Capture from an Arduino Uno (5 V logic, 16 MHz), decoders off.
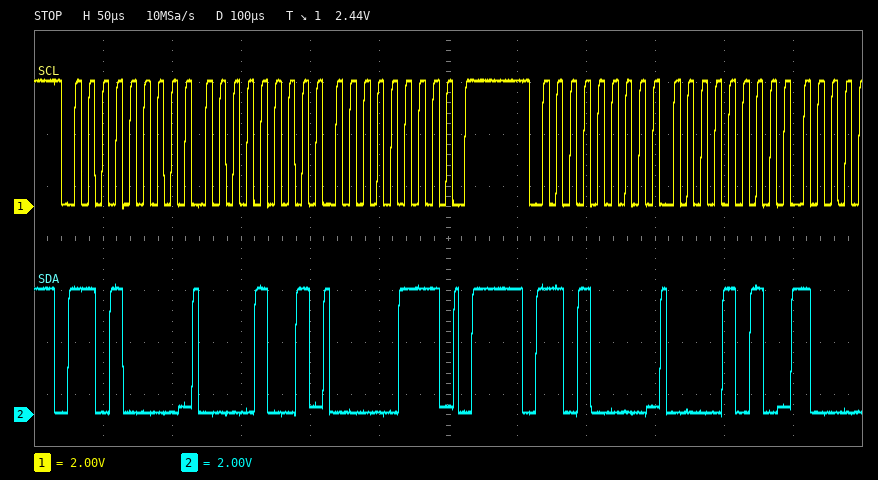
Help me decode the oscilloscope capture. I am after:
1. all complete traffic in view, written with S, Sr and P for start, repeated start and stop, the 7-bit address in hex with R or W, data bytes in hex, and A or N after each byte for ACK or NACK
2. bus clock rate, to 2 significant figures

S 68W A 09 A 07 A P S 68W A 0A A
100 kHz
